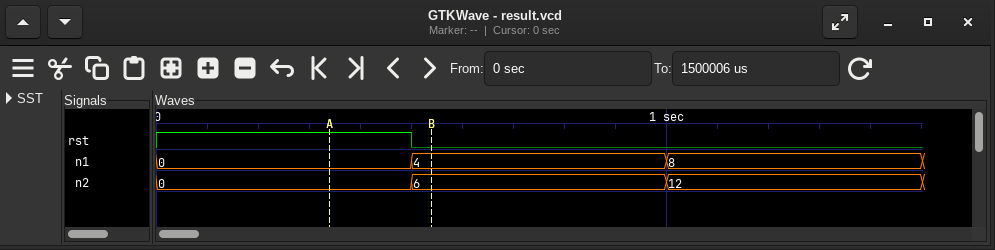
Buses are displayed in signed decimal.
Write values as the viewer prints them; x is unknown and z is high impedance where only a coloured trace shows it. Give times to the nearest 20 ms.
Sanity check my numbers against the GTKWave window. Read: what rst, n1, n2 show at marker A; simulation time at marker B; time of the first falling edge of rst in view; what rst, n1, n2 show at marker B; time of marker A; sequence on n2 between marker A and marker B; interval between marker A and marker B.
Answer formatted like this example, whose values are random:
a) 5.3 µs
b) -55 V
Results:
a) rst=1, n1=0, n2=0
b) 540 ms
c) 500 ms
d) rst=0, n1=4, n2=6
e) 340 ms
f) 0, 6
g) 200 ms
